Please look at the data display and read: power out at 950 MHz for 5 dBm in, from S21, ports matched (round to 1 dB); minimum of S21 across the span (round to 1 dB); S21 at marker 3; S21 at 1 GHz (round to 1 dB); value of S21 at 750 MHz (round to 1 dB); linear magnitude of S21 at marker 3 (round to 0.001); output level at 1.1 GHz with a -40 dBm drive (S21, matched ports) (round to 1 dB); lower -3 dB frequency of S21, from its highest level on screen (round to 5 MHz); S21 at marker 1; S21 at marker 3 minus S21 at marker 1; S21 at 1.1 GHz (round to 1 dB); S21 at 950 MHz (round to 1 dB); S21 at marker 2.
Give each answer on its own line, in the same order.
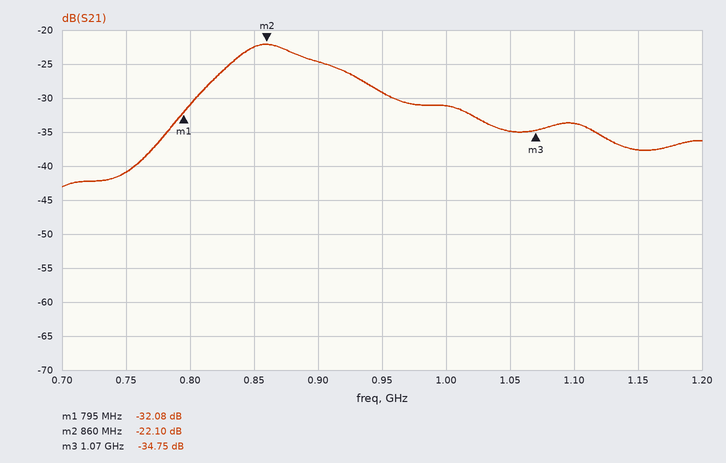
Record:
-24 dBm
-43 dB
-34.75 dB
-31 dB
-41 dB
0.018
-74 dBm
830 MHz
-32.08 dB
-2.67 dB
-34 dB
-29 dB
-22.10 dB
